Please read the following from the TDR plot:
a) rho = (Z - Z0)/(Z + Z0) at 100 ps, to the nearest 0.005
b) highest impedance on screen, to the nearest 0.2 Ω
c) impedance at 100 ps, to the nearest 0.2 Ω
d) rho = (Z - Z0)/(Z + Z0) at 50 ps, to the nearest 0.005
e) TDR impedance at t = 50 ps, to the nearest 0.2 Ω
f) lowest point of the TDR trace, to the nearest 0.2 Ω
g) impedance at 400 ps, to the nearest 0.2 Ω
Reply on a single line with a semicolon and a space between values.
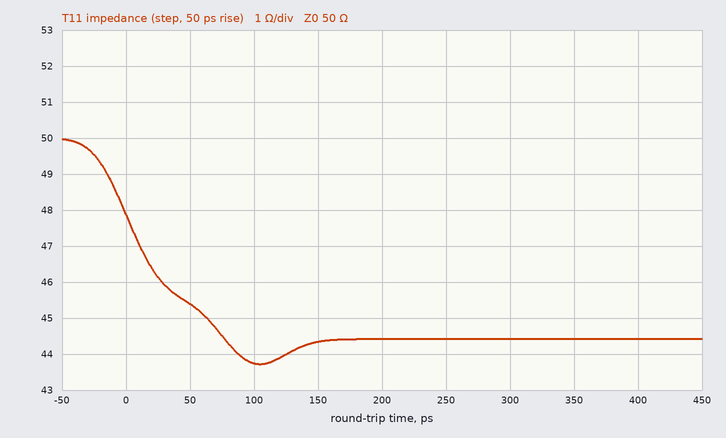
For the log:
-0.065; 50.0 Ω; 43.8 Ω; -0.050; 45.4 Ω; 43.8 Ω; 44.4 Ω
